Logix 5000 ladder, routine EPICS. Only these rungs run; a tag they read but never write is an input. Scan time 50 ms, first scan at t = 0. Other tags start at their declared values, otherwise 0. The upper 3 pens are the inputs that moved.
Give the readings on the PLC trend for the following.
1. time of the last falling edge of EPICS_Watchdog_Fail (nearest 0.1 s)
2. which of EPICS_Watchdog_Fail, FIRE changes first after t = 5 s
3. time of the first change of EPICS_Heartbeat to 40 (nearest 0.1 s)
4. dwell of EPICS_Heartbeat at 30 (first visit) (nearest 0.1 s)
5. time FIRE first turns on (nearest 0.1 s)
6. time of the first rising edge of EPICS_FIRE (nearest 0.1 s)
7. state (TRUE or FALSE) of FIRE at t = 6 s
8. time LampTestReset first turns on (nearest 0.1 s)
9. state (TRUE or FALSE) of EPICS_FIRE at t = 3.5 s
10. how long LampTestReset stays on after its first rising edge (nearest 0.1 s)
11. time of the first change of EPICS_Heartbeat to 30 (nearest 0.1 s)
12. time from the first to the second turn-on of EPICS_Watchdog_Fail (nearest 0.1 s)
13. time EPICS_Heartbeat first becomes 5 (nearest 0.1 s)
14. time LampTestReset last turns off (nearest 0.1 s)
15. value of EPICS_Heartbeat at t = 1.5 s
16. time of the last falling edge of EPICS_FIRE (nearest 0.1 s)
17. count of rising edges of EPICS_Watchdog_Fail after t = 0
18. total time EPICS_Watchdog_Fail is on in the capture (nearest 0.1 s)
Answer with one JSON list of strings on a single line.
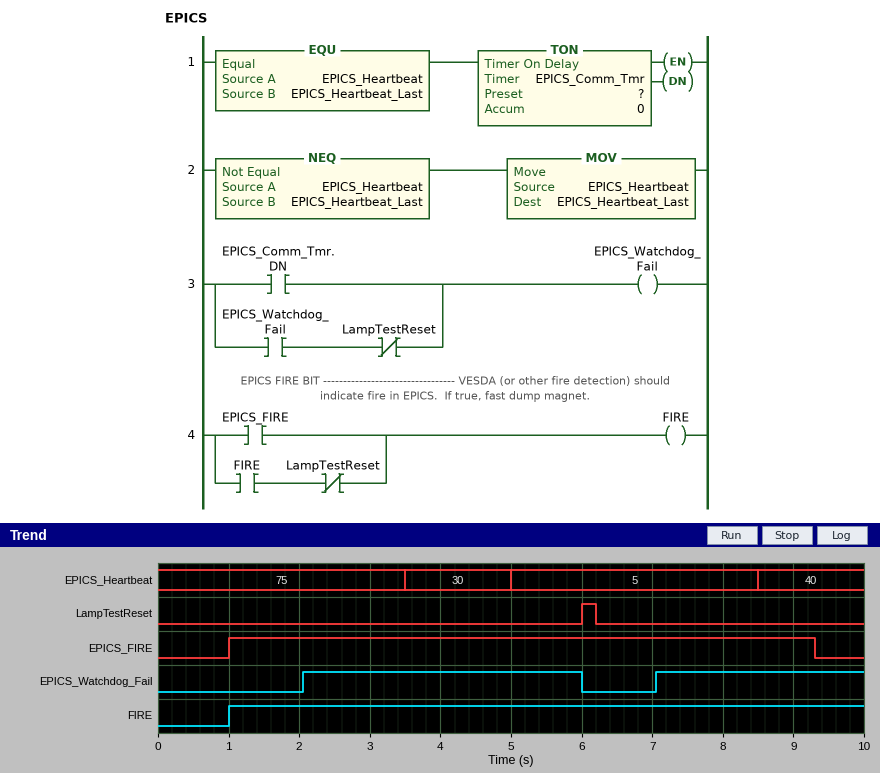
["6.0 s", "EPICS_Watchdog_Fail", "8.5 s", "1.5 s", "1.0 s", "1.0 s", "TRUE", "6.0 s", "TRUE", "0.2 s", "3.5 s", "5.0 s", "5.0 s", "6.2 s", "75", "9.3 s", "2", "6.9 s"]
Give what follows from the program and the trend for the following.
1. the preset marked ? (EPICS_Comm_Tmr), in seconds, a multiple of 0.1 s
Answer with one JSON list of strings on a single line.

["2.0 s"]
